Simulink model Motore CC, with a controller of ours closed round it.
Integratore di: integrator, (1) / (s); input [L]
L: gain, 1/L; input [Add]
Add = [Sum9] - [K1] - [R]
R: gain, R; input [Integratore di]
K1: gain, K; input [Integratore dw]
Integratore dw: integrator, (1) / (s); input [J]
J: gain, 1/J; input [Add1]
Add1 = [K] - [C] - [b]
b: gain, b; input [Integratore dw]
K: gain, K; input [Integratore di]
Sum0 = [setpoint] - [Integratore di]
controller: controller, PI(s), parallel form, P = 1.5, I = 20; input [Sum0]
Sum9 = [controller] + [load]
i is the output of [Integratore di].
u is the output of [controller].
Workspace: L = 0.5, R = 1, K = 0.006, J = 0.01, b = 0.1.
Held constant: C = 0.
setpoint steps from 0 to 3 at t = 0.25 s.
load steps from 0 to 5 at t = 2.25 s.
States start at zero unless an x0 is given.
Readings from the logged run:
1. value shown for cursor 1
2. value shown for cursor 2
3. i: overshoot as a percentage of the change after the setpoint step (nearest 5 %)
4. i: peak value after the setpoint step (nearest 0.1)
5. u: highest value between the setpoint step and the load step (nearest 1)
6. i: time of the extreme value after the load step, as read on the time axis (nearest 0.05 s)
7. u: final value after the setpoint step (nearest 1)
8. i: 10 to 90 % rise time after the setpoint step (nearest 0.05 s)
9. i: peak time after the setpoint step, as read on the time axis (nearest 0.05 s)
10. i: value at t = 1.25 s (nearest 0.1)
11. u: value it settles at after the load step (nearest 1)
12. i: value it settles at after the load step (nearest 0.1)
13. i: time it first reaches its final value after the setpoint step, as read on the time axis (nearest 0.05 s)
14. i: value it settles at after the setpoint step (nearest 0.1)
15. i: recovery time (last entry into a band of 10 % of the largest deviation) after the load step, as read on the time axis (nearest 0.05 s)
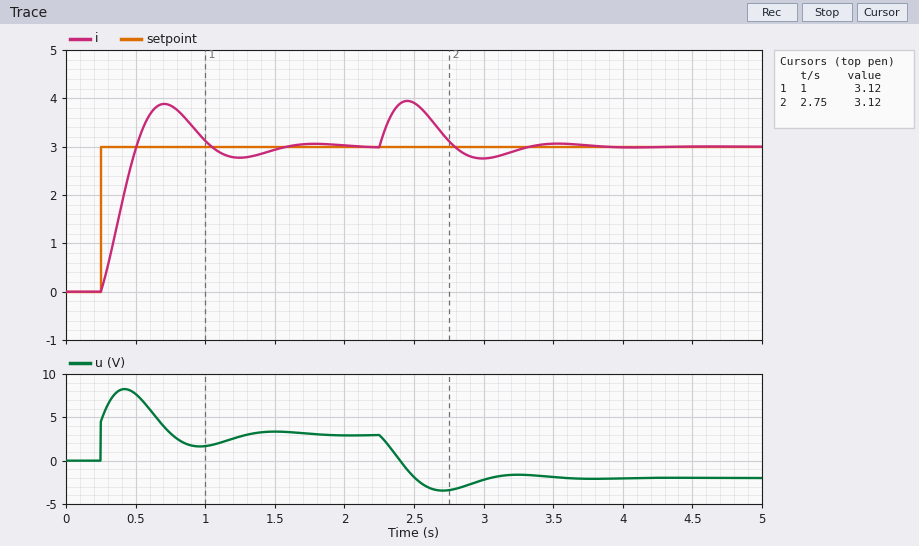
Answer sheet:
3.12
3.12
30 %
3.9
8
2.45 s
3
0.20 s
0.70 s
2.8
-2
3.0
0.50 s
3.0
3.20 s
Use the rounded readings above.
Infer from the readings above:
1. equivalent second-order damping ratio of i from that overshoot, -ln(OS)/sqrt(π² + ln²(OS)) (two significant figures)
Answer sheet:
0.36
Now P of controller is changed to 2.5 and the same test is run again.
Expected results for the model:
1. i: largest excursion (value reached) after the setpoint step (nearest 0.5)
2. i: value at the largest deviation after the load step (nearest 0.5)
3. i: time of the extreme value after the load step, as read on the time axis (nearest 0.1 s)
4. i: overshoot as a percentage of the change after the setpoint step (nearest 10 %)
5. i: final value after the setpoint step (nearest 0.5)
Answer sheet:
3.5
4.0
2.4 s
20 %
3.0
